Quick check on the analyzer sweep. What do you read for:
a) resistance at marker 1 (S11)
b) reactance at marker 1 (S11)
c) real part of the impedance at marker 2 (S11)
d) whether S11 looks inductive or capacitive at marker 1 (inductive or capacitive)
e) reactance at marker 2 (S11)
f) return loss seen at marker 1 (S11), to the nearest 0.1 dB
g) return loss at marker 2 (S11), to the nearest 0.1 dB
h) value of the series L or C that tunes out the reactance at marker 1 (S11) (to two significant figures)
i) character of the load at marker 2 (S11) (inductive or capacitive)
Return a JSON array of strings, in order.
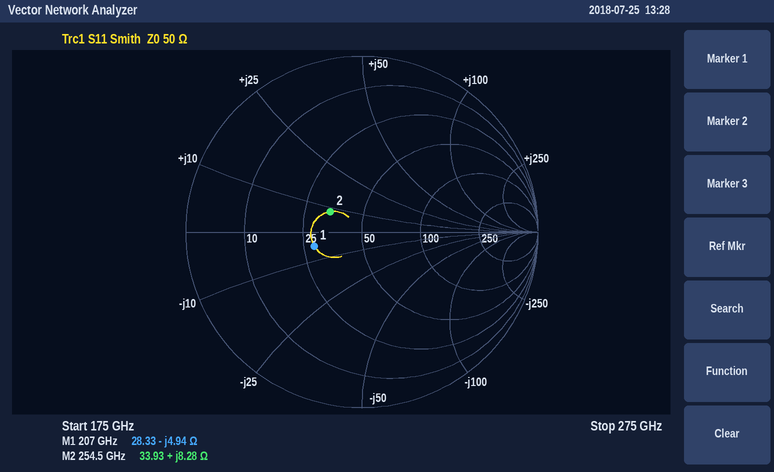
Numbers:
["28.33 Ω", "-4.94 Ω", "33.93 Ω", "capacitive", "+8.28 Ω", "11.0 dB", "13.4 dB", "3.8 pH", "inductive"]
